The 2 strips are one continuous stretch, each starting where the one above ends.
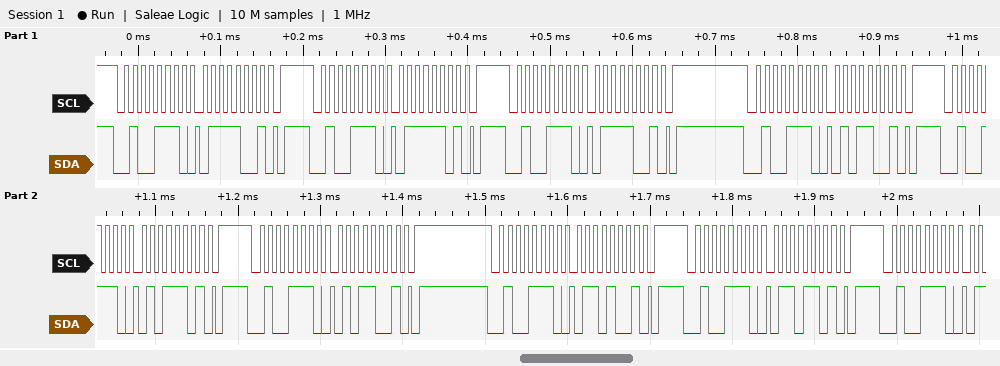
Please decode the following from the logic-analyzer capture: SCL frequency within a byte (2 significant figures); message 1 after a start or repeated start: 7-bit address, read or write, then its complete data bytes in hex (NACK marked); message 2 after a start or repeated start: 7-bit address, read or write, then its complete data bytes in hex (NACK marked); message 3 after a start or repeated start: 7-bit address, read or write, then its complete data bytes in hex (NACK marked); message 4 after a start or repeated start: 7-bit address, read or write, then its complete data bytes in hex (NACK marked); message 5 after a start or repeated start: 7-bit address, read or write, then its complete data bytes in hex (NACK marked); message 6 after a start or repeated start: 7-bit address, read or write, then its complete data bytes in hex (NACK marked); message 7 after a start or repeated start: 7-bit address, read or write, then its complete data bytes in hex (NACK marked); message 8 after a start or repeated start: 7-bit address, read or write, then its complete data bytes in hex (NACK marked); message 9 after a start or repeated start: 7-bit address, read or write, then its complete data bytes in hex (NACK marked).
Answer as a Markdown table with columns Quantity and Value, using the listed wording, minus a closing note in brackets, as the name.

| Quantity | Value |
|---|---|
| SCL frequency within a byte | 100 kHz |
| message 1 after a start or repeated start: 7-bit address, read or write, then its complete data bytes in hex | 0x27 write: 79 |
| message 2 after a start or repeated start: 7-bit address, read or write, then its complete data bytes in hex | 0x27 write: 7D |
| message 3 after a start or repeated start: 7-bit address, read or write, then its complete data bytes in hex | 0x27 write: 79 |
| message 4 after a start or repeated start: 7-bit address, read or write, then its complete data bytes in hex | 0x27 write: 59 |
| message 5 after a start or repeated start: 7-bit address, read or write, then its complete data bytes in hex | 0x27 write: 5D |
| message 6 after a start or repeated start: 7-bit address, read or write, then its complete data bytes in hex | 0x27 write: 59 |
| message 7 after a start or repeated start: 7-bit address, read or write, then its complete data bytes in hex | 0x27 write: 69 |
| message 8 after a start or repeated start: 7-bit address, read or write, then its complete data bytes in hex | 0x27 write: 6D |
| message 9 after a start or repeated start: 7-bit address, read or write, then its complete data bytes in hex | 0x27 write |
